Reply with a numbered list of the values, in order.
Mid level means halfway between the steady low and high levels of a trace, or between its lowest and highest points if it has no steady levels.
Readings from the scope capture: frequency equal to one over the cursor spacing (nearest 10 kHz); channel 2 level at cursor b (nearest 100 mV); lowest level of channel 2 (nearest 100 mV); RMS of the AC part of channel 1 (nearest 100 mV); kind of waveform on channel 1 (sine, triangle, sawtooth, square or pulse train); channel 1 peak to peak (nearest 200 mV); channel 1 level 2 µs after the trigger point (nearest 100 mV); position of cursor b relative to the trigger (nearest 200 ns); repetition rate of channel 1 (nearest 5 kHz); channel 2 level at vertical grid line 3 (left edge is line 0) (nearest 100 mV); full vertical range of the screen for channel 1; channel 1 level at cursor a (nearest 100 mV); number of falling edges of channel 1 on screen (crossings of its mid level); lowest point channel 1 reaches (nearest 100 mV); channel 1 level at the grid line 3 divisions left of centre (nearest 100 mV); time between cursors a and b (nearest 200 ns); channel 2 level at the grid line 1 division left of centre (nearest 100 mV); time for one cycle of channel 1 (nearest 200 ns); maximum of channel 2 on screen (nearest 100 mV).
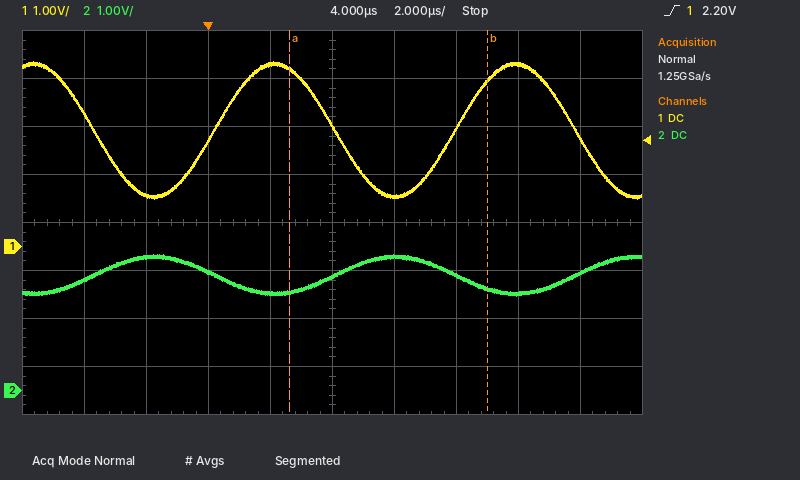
1. 160 kHz
2. 2.1 V
3. 2.0 V
4. 1.0 V
5. sine
6. 2.8 V
7. 3.8 V
8. +9.0 µs
9. 130 kHz
10. 2.5 V
11. 8 V
12. 3.7 V
13. 3
14. 1.0 V
15. 1.1 V
16. 6.4 µs
17. 2.0 V
18. 7.8 µs
19. 2.8 V
